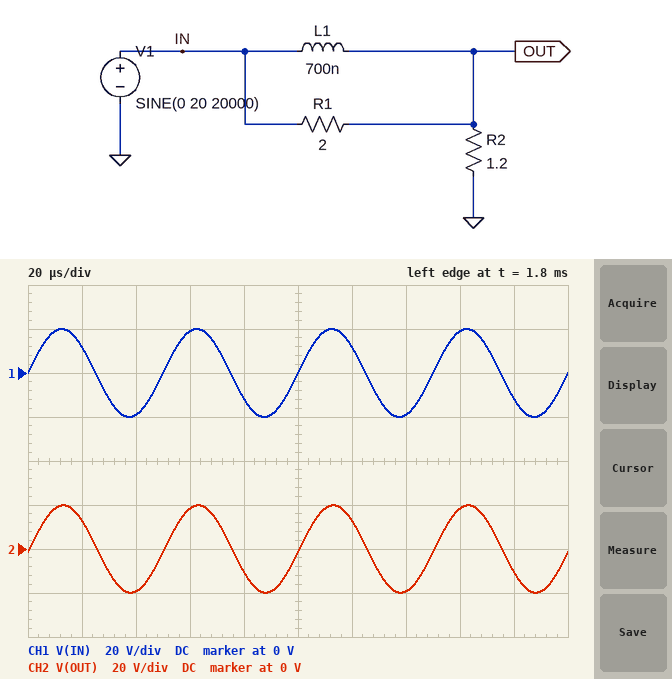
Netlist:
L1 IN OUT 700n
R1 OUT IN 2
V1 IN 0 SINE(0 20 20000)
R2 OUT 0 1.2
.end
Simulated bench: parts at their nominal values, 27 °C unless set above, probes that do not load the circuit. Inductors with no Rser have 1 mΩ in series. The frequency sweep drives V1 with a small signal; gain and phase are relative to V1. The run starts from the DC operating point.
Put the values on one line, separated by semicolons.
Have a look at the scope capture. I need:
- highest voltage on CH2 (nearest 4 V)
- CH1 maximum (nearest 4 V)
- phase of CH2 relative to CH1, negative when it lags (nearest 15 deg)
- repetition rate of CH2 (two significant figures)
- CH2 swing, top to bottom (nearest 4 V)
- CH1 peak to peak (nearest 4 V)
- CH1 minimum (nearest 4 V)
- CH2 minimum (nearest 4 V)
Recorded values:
20 V; 20 V; 0 deg; 20 kHz; 40 V; 40 V; -20 V; -20 V
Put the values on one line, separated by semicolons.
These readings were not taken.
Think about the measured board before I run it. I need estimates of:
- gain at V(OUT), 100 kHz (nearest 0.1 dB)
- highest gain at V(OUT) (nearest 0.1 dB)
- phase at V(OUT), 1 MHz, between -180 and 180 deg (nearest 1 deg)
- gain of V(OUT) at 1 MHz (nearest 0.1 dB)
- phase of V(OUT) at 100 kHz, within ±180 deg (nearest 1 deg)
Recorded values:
-1.1 dB; 0 dB; -15 deg; -7.8 dB; -18 deg
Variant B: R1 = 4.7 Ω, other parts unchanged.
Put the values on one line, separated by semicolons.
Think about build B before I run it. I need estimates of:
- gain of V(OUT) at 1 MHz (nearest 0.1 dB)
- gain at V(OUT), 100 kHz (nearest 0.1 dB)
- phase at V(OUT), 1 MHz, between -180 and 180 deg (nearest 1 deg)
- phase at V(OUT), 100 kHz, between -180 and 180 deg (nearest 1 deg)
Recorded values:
-10.7 dB; -0.8 dB; -35 deg; -19 deg
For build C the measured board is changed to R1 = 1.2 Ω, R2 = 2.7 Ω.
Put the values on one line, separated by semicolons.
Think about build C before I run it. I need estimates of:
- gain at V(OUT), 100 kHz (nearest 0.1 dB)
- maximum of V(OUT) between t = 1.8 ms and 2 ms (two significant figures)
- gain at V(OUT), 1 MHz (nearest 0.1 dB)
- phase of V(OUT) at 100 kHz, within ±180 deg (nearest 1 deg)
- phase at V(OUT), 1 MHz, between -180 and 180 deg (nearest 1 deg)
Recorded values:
-0.5 dB; 20 V; -3.0 dB; -8 deg; -5 deg
